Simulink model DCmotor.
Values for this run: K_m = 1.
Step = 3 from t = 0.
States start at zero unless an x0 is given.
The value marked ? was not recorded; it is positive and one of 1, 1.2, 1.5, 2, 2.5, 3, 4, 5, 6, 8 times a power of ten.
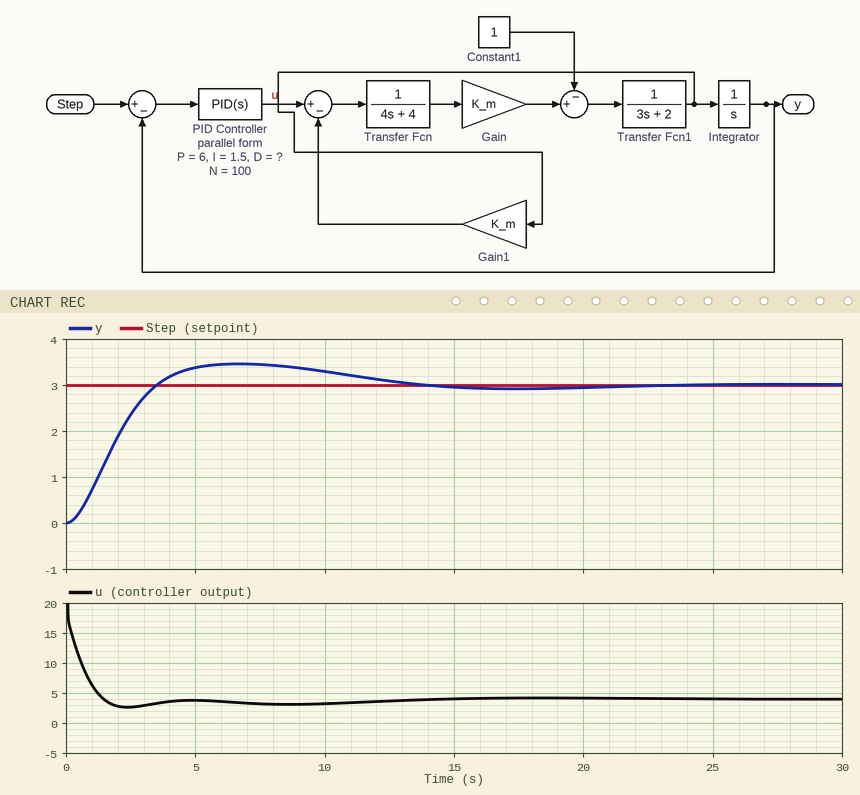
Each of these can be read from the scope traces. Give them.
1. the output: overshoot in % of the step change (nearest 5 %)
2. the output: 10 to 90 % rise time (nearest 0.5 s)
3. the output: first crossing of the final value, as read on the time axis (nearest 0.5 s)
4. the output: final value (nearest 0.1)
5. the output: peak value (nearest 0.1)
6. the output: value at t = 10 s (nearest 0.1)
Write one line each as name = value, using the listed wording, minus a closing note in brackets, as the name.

the output: overshoot in % of the step change = 15 %
the output: 10 to 90 % rise time = 2.5 s
the output: first crossing of the final value, as read on the time axis = 3.5 s
the output: final value = 3.0
the output: peak value = 3.5
the output: value at t = 10 s = 3.3
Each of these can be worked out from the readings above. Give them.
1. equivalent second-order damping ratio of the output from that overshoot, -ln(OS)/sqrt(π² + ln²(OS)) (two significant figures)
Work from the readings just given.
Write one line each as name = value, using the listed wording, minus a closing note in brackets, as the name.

equivalent second-order damping ratio of the output from that overshoot, -ln(OS)/sqrt(π² + ln²(OS)) = 0.52
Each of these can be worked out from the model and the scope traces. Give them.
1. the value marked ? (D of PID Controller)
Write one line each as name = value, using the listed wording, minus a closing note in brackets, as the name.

the value marked ? = 10
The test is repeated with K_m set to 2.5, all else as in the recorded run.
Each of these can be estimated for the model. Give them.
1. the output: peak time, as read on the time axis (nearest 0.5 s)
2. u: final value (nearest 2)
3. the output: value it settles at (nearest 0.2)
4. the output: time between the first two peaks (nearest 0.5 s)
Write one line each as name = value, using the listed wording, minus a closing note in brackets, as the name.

the output: peak time, as read on the time axis = 2.5 s
u: final value = 2
the output: value it settles at = 3.0
the output: time between the first two peaks = 4.0 s
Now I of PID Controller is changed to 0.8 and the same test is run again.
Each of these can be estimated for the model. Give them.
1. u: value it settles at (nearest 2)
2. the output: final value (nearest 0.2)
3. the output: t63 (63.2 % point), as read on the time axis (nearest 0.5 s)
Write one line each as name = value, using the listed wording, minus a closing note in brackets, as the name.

u: value it settles at = 4
the output: final value = 3.0
the output: t63 (63.2 % point), as read on the time axis = 2.0 s
